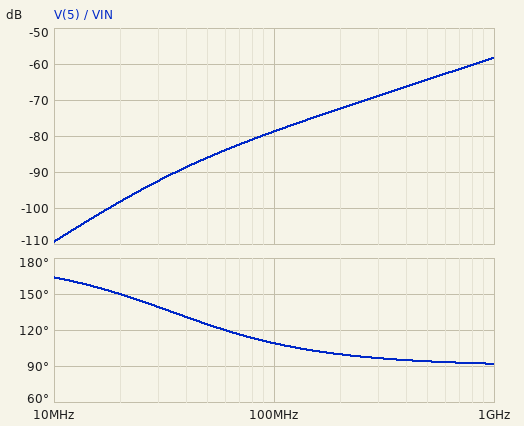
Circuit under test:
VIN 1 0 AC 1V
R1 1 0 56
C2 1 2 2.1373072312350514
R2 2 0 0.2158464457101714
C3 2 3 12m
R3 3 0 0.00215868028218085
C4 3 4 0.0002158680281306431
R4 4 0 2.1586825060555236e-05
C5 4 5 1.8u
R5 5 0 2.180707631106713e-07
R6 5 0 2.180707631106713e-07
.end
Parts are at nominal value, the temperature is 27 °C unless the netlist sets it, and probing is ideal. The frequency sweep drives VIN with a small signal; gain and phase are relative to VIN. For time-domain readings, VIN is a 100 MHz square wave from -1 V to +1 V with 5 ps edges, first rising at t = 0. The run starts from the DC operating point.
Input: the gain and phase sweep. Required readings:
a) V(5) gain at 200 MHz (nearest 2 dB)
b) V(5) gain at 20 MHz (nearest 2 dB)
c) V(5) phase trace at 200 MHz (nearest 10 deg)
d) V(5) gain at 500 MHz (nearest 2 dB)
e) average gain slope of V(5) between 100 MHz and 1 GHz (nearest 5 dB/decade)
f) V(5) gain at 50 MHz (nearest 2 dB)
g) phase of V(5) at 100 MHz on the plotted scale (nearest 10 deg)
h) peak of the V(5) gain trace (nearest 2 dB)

-72 dB
-98 dB
100 deg
-64 dB
20 dB/decade
-86 dB
110 deg
-58 dB
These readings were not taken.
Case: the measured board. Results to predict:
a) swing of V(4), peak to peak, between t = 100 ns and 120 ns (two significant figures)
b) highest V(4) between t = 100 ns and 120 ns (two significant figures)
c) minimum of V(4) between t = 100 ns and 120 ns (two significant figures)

3.0 V
1.5 V
-1.5 V
